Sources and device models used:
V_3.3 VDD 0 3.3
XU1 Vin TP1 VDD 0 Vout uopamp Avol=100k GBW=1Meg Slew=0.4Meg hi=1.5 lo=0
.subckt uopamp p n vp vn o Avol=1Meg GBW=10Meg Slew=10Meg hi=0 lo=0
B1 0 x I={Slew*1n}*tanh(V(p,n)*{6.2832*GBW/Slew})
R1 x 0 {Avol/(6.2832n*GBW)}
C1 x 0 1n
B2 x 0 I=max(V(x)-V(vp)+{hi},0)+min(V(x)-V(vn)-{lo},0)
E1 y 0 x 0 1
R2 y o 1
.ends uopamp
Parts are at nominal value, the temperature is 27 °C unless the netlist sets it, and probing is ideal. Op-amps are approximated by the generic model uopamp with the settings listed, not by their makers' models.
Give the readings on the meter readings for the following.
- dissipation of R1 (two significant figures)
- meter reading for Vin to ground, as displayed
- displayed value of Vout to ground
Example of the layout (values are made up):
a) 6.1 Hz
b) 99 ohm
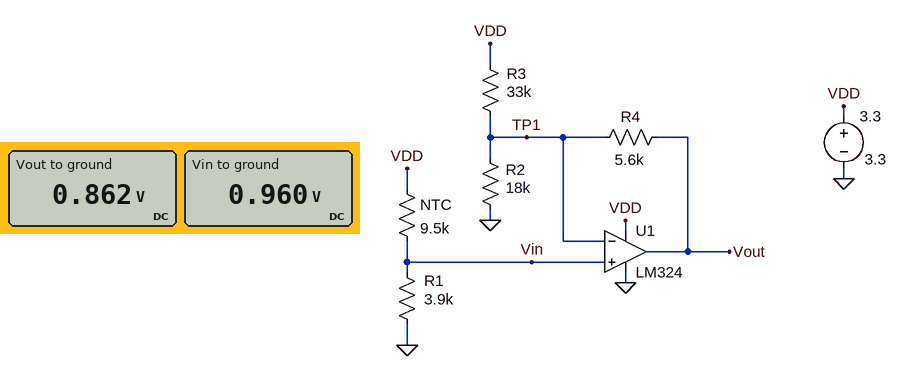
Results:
a) 240 µW
b) 0.960 V
c) 0.862 V
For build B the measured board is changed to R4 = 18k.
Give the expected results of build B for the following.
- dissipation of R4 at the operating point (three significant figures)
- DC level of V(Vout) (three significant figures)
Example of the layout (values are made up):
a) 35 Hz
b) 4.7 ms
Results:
a) 5.54 µW
b) 645 mV
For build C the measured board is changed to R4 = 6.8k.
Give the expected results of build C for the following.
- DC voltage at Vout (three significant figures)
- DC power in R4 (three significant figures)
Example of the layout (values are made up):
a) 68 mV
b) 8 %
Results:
a) 841 mV
b) 2.09 µW
